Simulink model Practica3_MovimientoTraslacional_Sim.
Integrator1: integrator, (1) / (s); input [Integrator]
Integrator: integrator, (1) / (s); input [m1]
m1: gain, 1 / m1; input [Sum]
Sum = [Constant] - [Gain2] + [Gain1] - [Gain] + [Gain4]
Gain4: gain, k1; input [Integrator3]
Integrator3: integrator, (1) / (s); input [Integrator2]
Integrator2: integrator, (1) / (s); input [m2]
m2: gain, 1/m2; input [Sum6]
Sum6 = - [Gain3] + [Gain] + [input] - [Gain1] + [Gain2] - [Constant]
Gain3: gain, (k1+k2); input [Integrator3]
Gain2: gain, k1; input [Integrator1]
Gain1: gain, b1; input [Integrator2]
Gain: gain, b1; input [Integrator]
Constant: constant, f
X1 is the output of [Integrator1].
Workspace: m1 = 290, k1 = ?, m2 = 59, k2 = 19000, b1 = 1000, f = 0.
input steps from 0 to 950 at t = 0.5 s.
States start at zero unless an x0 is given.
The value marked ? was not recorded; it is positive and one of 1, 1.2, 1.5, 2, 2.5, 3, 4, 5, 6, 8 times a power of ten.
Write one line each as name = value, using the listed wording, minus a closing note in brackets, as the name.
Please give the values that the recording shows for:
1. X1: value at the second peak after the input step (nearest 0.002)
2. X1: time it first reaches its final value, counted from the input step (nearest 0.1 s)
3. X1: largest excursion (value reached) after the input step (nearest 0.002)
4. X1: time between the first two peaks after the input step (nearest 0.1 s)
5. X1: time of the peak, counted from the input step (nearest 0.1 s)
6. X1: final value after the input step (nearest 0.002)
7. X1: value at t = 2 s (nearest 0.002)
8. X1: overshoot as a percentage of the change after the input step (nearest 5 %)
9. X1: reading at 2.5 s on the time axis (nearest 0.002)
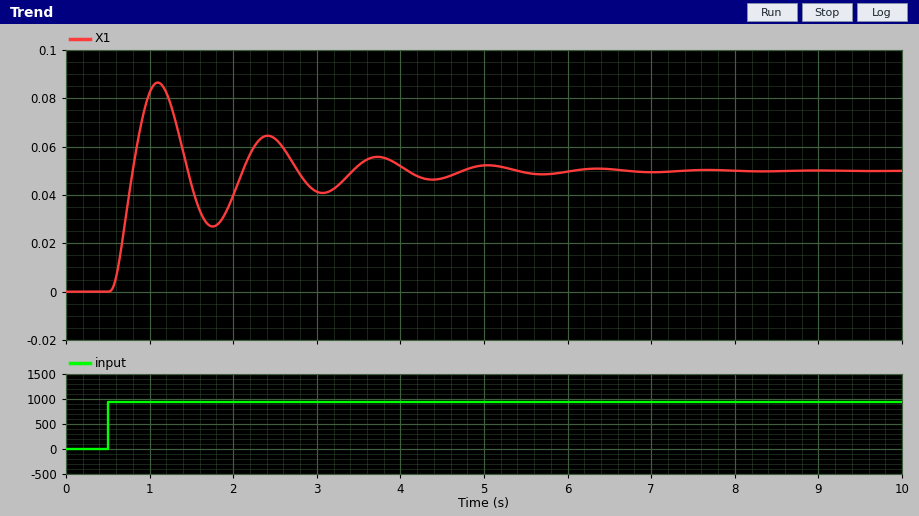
X1: value at the second peak after the input step = 0.064
X1: time it first reaches its final value, counted from the input step = 0.3 s
X1: largest excursion (value reached) after the input step = 0.086
X1: time between the first two peaks after the input step = 1.3 s
X1: time of the peak, counted from the input step = 0.6 s
X1: final value after the input step = 0.050
X1: value at t = 2 s = 0.040
X1: overshoot as a percentage of the change after the input step = 75 %
X1: reading at 2.5 s on the time axis = 0.064
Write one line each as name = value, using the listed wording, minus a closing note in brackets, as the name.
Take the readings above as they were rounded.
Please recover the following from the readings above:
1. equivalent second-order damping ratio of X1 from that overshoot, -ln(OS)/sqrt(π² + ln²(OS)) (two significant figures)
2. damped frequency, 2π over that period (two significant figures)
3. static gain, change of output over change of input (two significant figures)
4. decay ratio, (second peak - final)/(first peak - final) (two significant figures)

equivalent second-order damping ratio of X1 from that overshoot, -ln(OS)/sqrt(π² + ln²(OS)) = 0.091
damped frequency, 2π over that period = 4.8 rad/s
static gain, change of output over change of input = 0.000053
decay ratio, (second peak - final)/(first peak - final) = 0.39
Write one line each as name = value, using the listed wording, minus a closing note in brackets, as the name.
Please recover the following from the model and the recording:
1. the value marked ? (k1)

the value marked ? = 10000
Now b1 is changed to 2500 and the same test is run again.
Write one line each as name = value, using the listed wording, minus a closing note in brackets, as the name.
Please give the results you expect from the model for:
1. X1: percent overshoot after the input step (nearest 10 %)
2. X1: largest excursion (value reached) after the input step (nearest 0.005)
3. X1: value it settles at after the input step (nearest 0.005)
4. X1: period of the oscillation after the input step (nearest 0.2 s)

X1: percent overshoot after the input step = 60 %
X1: largest excursion (value reached) after the input step = 0.080
X1: value it settles at after the input step = 0.050
X1: period of the oscillation after the input step = 1.2 s
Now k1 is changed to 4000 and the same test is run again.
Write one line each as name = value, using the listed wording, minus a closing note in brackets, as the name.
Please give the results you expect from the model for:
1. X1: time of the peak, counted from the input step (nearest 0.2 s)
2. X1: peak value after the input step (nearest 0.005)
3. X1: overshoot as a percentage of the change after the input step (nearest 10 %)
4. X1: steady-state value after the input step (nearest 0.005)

X1: time of the peak, counted from the input step = 0.8 s
X1: peak value after the input step = 0.075
X1: overshoot as a percentage of the change after the input step = 50 %
X1: steady-state value after the input step = 0.050
